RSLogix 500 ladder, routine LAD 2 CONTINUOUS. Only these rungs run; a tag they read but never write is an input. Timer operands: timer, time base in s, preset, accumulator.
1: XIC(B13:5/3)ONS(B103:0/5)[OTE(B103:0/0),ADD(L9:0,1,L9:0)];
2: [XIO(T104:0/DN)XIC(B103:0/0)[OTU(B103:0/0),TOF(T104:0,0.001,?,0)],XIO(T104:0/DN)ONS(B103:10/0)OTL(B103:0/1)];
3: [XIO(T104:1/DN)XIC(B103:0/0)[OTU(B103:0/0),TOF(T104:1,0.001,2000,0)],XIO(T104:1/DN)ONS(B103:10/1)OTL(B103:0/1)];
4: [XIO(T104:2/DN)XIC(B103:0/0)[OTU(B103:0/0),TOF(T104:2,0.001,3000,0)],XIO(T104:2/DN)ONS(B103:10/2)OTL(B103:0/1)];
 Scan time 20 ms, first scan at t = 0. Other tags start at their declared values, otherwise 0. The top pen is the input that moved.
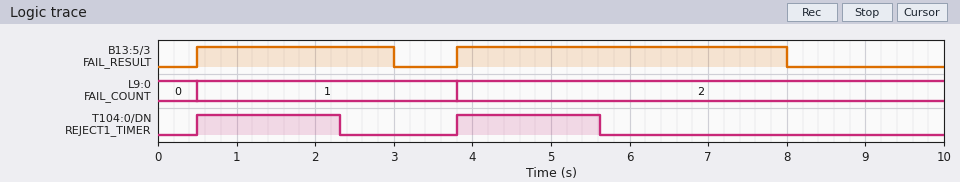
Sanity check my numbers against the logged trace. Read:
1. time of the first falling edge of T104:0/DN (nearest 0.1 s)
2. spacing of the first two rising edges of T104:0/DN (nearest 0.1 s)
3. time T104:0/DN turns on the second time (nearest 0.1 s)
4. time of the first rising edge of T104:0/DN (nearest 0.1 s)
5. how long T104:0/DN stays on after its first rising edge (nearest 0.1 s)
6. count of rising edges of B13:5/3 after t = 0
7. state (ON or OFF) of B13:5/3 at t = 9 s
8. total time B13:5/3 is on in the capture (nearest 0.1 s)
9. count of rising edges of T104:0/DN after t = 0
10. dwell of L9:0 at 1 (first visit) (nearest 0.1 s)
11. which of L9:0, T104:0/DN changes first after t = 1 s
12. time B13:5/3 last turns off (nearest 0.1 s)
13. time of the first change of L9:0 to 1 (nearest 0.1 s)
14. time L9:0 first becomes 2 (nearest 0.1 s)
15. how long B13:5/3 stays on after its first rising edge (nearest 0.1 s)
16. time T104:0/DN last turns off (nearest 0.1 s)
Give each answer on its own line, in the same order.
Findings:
2.3 s
3.3 s
3.8 s
0.5 s
1.8 s
2
OFF
6.7 s
2
3.3 s
T104:0/DN
8.0 s
0.5 s
3.8 s
2.5 s
5.6 s
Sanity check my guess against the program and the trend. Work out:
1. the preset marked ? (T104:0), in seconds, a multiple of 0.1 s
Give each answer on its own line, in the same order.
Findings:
1.8 s
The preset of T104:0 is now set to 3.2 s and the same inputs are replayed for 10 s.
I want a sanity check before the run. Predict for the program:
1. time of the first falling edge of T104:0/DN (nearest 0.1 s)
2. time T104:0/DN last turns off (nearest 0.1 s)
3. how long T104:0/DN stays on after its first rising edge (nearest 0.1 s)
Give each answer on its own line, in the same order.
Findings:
3.7 s
7.0 s
3.2 s
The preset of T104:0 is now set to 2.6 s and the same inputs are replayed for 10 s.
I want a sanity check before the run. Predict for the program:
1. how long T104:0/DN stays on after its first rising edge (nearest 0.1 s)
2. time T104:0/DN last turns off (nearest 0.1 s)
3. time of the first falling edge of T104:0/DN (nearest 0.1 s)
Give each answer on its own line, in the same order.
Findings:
2.6 s
6.4 s
3.1 s
